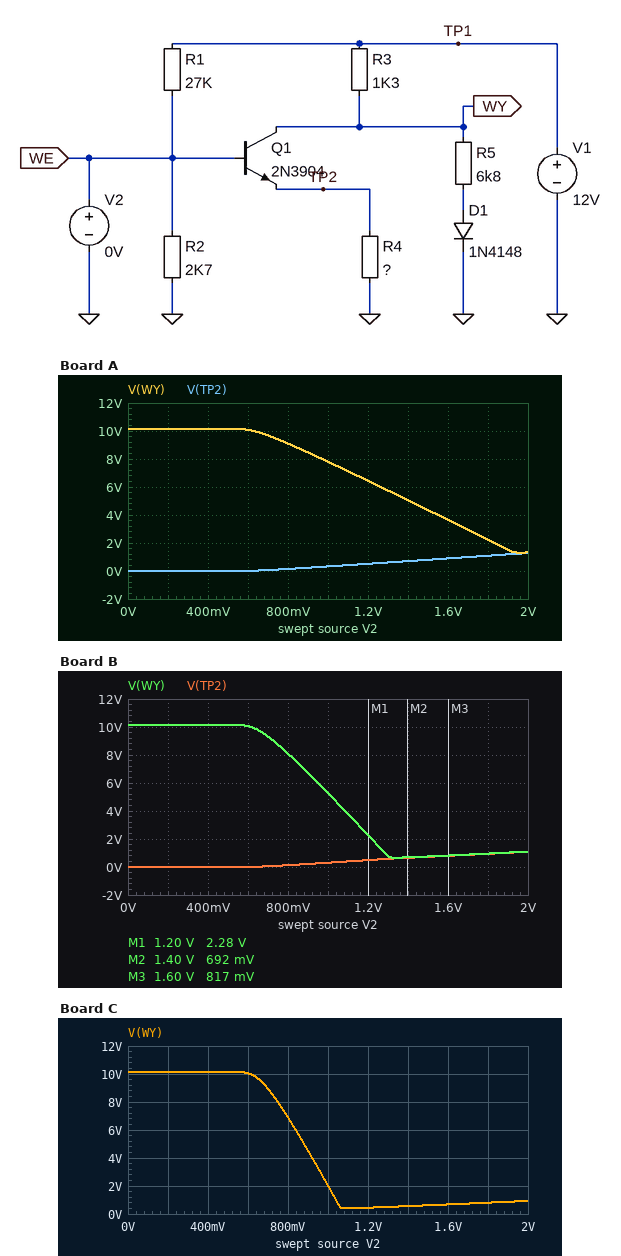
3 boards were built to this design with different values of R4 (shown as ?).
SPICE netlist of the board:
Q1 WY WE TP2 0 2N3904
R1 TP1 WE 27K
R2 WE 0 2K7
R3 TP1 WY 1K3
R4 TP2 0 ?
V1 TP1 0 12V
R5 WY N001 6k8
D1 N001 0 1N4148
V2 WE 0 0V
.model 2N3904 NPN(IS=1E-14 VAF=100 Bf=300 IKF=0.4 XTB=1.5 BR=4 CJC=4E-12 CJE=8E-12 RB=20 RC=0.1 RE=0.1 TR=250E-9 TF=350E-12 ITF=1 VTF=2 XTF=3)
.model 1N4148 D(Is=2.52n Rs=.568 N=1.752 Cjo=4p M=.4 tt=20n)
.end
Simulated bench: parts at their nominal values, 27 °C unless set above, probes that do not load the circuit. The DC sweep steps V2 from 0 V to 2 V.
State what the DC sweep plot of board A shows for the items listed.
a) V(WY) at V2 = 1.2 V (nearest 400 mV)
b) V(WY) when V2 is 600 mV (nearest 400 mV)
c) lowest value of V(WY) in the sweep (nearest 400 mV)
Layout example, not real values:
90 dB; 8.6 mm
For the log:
6.4 V; 10.0 V; 1.2 V
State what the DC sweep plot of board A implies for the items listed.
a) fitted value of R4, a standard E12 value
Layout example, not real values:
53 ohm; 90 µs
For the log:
150 Ω
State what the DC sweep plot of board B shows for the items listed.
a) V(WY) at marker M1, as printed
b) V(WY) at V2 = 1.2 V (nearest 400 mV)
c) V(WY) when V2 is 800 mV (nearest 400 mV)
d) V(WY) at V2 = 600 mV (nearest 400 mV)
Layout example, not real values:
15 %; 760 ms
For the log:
2.28 V; 2.4 V; 8.0 V; 10.0 V
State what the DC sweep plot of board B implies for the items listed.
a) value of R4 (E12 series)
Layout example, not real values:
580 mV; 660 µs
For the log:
68 Ω
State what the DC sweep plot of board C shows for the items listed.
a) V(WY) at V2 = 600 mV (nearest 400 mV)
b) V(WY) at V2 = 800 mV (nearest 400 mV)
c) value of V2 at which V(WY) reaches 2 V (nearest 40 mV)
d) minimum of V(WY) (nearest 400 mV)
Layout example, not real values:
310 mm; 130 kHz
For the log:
10.0 V; 6.8 V; 1.00 V; 400 mV
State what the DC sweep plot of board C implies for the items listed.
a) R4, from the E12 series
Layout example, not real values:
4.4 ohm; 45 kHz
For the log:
39 Ω
